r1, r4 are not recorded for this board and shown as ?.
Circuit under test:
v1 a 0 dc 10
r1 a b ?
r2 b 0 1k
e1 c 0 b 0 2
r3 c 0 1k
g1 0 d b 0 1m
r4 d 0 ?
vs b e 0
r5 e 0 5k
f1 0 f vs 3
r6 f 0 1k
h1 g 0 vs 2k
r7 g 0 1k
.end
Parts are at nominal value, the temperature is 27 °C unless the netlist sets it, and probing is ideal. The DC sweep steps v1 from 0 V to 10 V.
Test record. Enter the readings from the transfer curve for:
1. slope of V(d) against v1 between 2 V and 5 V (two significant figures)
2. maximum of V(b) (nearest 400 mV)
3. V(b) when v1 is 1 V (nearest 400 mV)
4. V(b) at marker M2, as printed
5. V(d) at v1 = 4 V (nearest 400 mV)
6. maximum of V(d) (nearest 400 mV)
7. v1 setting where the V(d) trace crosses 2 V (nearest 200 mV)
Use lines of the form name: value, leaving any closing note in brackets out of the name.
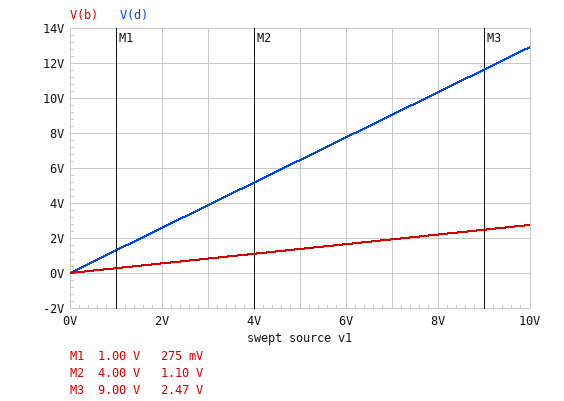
slope of V(d) against v1 between 2 V and 5 V: 1.3 V/V
maximum of V(b): 2.8 V
V(b) when v1 is 1 V: 400 mV
V(b) at marker M2, as printed: 1.10 V
V(d) at v1 = 4 V: 5.2 V
maximum of V(d): 12.8 V
v1 setting where the V(d) trace crosses 2 V: 1.6 V
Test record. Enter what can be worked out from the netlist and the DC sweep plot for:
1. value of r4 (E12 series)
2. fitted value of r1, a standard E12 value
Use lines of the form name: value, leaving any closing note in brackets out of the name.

value of r4: 4.7 kΩ
fitted value of r1, a standard E12 value: 2.2 kΩ
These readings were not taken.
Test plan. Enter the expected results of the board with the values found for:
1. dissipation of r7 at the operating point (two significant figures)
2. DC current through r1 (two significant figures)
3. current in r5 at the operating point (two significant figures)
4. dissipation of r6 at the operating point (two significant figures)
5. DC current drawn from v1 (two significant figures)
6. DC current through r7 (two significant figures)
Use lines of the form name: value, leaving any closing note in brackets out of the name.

dissipation of r7 at the operating point: 1.2 mW
DC current through r1: 3.3 mA
current in r5 at the operating point: 550 µA
dissipation of r6 at the operating point: 2.7 mW
DC current drawn from v1: 3.3 mA
DC current through r7: 1.1 mA
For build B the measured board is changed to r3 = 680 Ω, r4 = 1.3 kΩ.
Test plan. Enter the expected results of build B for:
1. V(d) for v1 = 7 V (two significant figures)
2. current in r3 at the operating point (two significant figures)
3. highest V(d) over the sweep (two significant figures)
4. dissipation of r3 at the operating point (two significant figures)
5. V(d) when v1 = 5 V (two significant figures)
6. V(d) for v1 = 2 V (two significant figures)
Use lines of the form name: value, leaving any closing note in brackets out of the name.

V(d) for v1 = 7 V: 2.5 V
current in r3 at the operating point: 8.1 mA
highest V(d) over the sweep: 3.6 V
dissipation of r3 at the operating point: 44 mW
V(d) when v1 = 5 V: 1.8 V
V(d) for v1 = 2 V: 710 mV
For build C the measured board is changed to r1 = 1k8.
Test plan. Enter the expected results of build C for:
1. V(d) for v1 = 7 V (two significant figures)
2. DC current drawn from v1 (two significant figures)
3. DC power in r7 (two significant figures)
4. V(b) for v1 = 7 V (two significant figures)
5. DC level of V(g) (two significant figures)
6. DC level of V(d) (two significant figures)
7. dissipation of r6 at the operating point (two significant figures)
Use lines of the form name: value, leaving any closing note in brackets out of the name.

V(d) for v1 = 7 V: 10 V
DC current drawn from v1: 3.8 mA
DC power in r7: 1.6 mW
V(b) for v1 = 7 V: 2.2 V
DC level of V(g): 1.3 V
DC level of V(d): 15 V
dissipation of r6 at the operating point: 3.6 mW
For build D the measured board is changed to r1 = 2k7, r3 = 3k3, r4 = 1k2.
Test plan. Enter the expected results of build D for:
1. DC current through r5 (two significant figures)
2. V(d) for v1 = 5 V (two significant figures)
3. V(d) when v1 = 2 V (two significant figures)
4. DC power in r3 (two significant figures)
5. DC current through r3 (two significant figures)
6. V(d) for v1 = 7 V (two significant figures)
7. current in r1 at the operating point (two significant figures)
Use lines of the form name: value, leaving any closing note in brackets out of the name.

DC current through r5: 470 µA
V(d) for v1 = 5 V: 1.4 V
V(d) when v1 = 2 V: 570 mV
DC power in r3: 6.7 mW
DC current through r3: 1.4 mA
V(d) for v1 = 7 V: 2.0 V
current in r1 at the operating point: 2.8 mA
